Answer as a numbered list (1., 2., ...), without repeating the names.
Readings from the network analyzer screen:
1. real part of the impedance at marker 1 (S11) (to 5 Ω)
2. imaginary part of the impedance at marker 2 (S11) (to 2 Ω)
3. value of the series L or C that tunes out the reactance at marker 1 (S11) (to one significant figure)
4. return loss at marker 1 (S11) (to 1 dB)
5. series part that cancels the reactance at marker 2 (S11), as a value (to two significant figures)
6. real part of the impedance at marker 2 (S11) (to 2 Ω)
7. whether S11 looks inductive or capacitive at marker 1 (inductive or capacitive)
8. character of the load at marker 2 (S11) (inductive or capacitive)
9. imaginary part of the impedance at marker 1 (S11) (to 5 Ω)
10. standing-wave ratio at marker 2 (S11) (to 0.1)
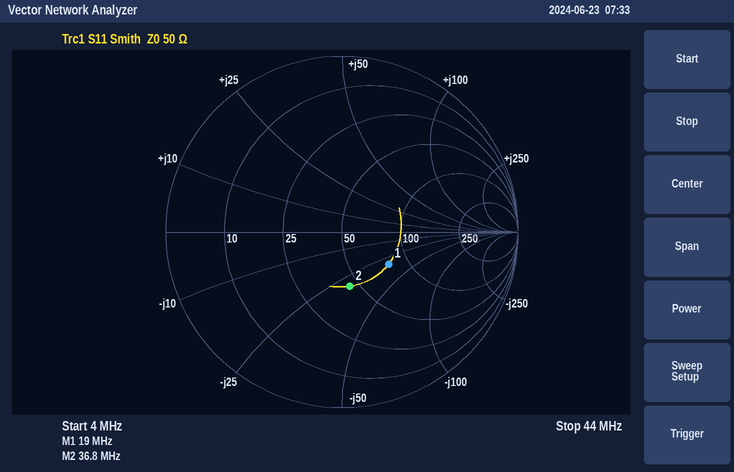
1. 80 Ω
2. -30 Ω
3. 300 nH
4. 10 dB
5. 130 nH
6. 44 Ω
7. capacitive
8. capacitive
9. -30 Ω
10. 1.9
